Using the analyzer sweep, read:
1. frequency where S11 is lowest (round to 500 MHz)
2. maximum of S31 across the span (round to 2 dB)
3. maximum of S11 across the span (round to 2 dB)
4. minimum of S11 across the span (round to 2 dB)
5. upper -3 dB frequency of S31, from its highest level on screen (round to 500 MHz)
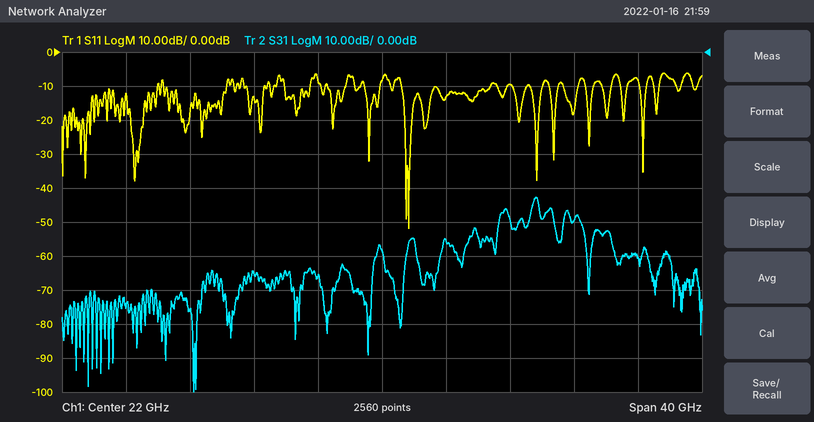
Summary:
23.5 GHz
-42 dB
-6 dB
-52 dB
32.0 GHz
